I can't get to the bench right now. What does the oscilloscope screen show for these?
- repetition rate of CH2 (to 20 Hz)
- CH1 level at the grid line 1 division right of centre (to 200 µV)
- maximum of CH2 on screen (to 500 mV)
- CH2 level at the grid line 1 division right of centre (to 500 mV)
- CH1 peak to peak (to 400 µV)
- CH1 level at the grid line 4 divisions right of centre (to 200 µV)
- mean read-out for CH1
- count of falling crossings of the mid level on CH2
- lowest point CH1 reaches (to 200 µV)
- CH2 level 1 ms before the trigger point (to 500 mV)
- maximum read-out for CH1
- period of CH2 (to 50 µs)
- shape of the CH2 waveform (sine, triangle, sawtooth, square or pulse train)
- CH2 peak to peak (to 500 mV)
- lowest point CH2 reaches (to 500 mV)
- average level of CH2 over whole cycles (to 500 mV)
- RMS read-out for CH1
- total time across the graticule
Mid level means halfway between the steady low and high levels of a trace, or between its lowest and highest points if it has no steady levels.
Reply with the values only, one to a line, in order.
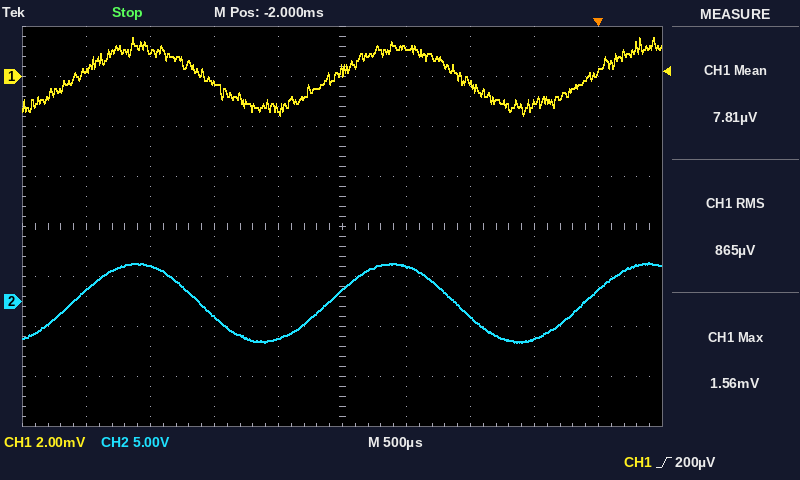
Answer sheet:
500 Hz
1.2 mV
4.0 V
3.5 V
3.2 mV
200 µV
7.81 µV
2
-1.6 mV
-1.5 V
1.56 mV
2.00 ms
sine
8.0 V
-4.0 V
0.0 V
865 µV
5 ms
